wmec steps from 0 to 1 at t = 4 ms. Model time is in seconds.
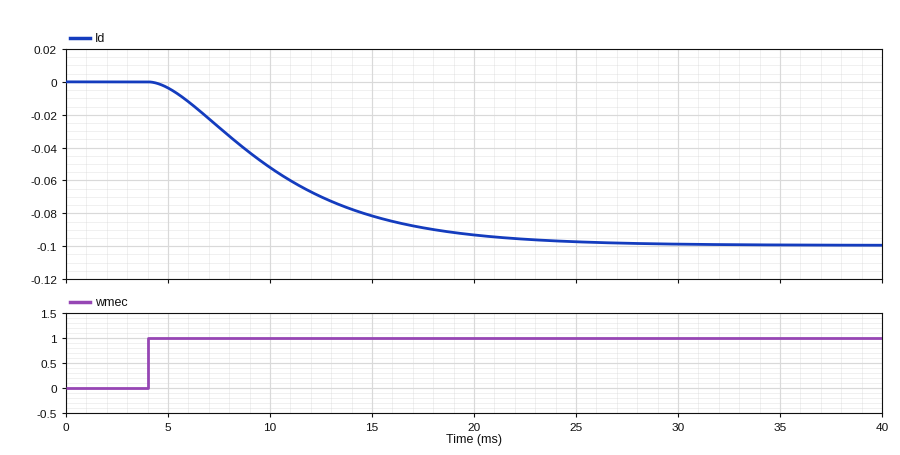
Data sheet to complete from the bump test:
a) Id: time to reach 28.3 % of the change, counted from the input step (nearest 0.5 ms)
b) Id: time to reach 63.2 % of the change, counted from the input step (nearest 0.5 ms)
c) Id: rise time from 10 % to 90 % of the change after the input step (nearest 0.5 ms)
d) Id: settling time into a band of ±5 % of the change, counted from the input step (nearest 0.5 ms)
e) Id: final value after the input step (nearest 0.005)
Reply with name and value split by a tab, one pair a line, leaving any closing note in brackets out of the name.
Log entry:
Id: time to reach 28.3 % of the change, counted from the input step	3.5 ms
Id: time to reach 63.2 % of the change, counted from the input step	7.5 ms
Id: rise time from 10 % to 90 % of the change after the input step	12.0 ms
Id: settling time into a band of ±5 % of the change, counted from the input step	17.0 ms
Id: final value after the input step	-0.100
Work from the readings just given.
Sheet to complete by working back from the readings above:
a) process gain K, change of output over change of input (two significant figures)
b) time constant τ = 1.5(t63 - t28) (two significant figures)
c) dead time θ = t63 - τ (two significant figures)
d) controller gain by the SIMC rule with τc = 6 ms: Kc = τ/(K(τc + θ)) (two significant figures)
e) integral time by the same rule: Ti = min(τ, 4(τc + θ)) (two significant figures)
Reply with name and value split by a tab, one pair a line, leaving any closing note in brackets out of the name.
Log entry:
process gain K, change of output over change of input	-0.10
time constant τ = 1.5(t63 - t28)	6.0 ms
dead time θ = t63 - τ	1.5 ms
controller gain by the SIMC rule with τc = 6 ms: Kc = τ/(K(τc + θ))	-8.0
integral time by the same rule: Ti = min(τ, 4(τc + θ))	6.0 ms
